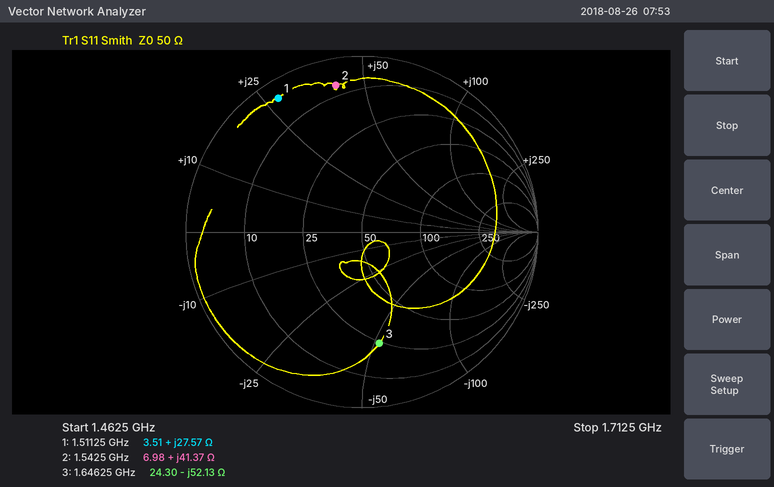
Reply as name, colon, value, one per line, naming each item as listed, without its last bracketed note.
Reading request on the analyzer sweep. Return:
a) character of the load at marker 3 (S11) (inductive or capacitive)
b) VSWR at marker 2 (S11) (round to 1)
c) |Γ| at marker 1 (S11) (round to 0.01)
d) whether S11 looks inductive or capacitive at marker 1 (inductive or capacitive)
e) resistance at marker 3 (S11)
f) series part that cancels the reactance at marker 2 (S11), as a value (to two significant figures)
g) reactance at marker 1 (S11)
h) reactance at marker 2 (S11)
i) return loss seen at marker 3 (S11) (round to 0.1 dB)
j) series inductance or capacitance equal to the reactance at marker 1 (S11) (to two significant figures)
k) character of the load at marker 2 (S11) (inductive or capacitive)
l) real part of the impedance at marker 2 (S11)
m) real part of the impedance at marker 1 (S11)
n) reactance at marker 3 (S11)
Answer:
character of the load at marker 3 (S11): capacitive
VSWR at marker 2 (S11): 12
|Γ| at marker 1 (S11): 0.90
whether S11 looks inductive or capacitive at marker 1: inductive
resistance at marker 3: 24.30 Ω
series part that cancels the reactance at marker 2 (S11), as a value: 2.5 pF
reactance at marker 1: +27.57 Ω
reactance at marker 2: +41.37 Ω
return loss seen at marker 3 (S11): 3.9 dB
series inductance or capacitance equal to the reactance at marker 1 (S11): 2.9 nH
character of the load at marker 2 (S11): inductive
real part of the impedance at marker 2: 6.98 Ω
real part of the impedance at marker 1: 3.51 Ω
reactance at marker 3: -52.13 Ω
